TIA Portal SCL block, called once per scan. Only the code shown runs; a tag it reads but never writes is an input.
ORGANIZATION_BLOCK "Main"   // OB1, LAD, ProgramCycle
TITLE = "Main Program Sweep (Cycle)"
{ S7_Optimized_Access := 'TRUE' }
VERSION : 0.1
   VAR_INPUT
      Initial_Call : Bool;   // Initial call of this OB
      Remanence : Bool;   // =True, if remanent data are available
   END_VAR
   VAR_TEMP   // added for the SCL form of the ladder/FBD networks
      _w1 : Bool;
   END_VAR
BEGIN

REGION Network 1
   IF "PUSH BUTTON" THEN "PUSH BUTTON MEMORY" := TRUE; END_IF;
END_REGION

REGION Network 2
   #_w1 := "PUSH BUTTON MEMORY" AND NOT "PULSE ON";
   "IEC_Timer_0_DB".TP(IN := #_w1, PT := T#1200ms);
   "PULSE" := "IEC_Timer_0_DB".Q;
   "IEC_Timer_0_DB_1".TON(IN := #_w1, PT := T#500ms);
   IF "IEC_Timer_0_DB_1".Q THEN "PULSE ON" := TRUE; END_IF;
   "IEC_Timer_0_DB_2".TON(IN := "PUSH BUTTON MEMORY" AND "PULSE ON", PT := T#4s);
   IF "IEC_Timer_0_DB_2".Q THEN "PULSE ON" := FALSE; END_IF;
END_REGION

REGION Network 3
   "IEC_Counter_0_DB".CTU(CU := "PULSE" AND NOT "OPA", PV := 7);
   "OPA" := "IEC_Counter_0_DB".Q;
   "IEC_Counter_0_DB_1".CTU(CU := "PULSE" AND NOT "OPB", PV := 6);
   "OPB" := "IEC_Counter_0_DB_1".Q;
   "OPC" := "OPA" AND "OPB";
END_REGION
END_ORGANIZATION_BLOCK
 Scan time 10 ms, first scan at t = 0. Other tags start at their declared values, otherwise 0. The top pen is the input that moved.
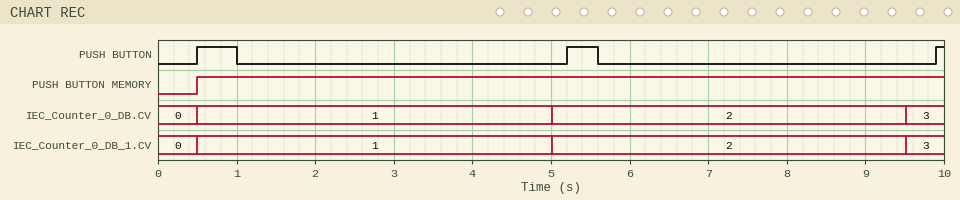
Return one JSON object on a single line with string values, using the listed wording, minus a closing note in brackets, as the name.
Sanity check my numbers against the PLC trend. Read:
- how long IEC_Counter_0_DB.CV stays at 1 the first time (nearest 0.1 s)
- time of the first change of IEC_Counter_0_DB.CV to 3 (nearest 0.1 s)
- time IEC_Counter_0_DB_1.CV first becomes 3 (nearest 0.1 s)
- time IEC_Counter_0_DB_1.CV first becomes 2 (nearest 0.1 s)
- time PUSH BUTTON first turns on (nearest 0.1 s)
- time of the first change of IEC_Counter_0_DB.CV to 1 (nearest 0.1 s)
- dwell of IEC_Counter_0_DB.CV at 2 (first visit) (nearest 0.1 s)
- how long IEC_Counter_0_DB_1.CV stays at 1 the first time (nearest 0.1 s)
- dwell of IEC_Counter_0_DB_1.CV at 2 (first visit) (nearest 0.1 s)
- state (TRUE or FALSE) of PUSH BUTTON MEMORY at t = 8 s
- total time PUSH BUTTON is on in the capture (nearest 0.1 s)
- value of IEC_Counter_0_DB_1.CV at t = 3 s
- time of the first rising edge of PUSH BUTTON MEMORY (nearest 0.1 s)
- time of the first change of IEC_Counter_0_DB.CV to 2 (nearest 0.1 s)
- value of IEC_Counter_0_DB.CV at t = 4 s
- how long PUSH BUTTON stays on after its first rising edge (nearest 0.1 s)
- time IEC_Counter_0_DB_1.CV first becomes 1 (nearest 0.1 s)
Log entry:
{"how long IEC_Counter_0_DB.CV stays at 1 the first time": "4.5 s", "time of the first change of IEC_Counter_0_DB.CV to 3": "9.5 s", "time IEC_Counter_0_DB_1.CV first becomes 3": "9.5 s", "time IEC_Counter_0_DB_1.CV first becomes 2": "5.0 s", "time PUSH BUTTON first turns on": "0.5 s", "time of the first change of IEC_Counter_0_DB.CV to 1": "0.5 s", "dwell of IEC_Counter_0_DB.CV at 2 (first visit)": "4.5 s", "how long IEC_Counter_0_DB_1.CV stays at 1 the first time": "4.5 s", "dwell of IEC_Counter_0_DB_1.CV at 2 (first visit)": "4.5 s", "state (TRUE or FALSE) of PUSH BUTTON MEMORY at t = 8 s": "TRUE", "total time PUSH BUTTON is on in the capture": "1.0 s", "value of IEC_Counter_0_DB_1.CV at t = 3 s": "1", "time of the first rising edge of PUSH BUTTON MEMORY": "0.5 s", "time of the first change of IEC_Counter_0_DB.CV to 2": "5.0 s", "value of IEC_Counter_0_DB.CV at t = 4 s": "1", "how long PUSH BUTTON stays on after its first rising edge": "0.5 s", "time IEC_Counter_0_DB_1.CV first becomes 1": "0.5 s"}
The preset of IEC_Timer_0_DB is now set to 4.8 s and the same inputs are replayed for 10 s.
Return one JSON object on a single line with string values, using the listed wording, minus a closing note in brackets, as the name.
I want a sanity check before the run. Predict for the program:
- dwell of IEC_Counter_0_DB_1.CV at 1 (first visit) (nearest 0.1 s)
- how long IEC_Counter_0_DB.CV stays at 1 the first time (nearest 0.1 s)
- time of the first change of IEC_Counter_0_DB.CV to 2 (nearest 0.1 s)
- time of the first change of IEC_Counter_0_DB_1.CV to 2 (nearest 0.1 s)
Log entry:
{"dwell of IEC_Counter_0_DB_1.CV at 1 (first visit)": "9.0 s", "how long IEC_Counter_0_DB.CV stays at 1 the first time": "9.0 s", "time of the first change of IEC_Counter_0_DB.CV to 2": "9.5 s", "time of the first change of IEC_Counter_0_DB_1.CV to 2": "9.5 s"}
